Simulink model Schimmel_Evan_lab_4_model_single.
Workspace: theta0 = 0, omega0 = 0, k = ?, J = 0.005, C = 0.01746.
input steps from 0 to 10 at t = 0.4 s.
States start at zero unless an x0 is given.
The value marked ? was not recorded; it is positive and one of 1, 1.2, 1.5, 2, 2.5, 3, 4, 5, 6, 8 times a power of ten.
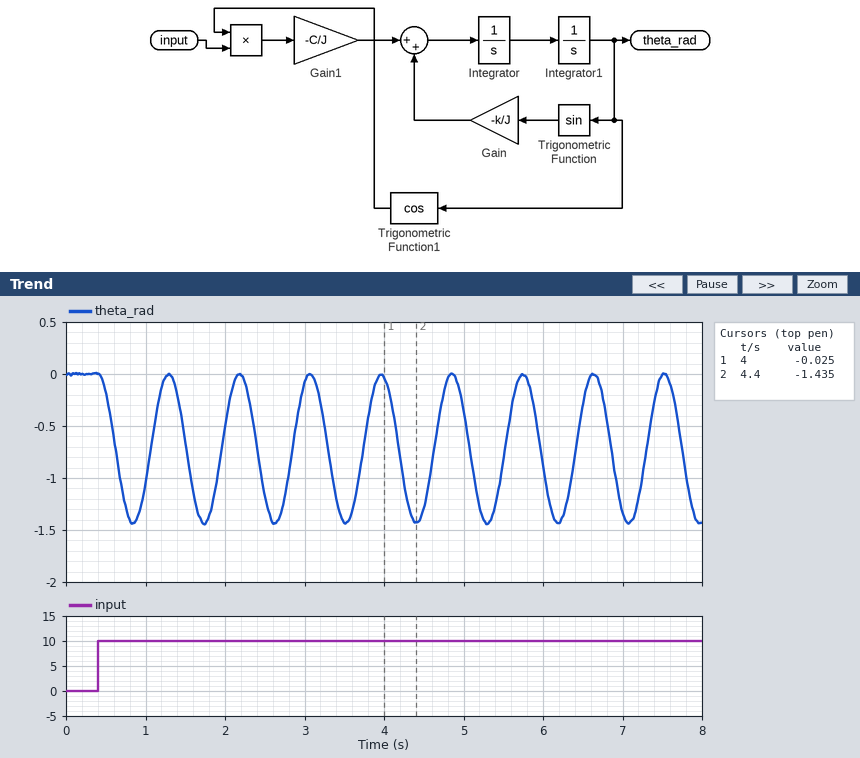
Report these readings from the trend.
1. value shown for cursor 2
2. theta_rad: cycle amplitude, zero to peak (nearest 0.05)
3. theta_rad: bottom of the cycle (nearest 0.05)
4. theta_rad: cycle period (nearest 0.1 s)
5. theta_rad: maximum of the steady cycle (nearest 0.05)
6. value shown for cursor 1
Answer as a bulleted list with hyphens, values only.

- -1.435
- 0.70
- -1.45
- 0.9 s
- 0.00
- -0.025
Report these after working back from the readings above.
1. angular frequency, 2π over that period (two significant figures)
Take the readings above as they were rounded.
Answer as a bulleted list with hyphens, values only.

- 7.0 rad/s
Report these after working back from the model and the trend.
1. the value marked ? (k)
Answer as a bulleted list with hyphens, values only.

- 0.2
